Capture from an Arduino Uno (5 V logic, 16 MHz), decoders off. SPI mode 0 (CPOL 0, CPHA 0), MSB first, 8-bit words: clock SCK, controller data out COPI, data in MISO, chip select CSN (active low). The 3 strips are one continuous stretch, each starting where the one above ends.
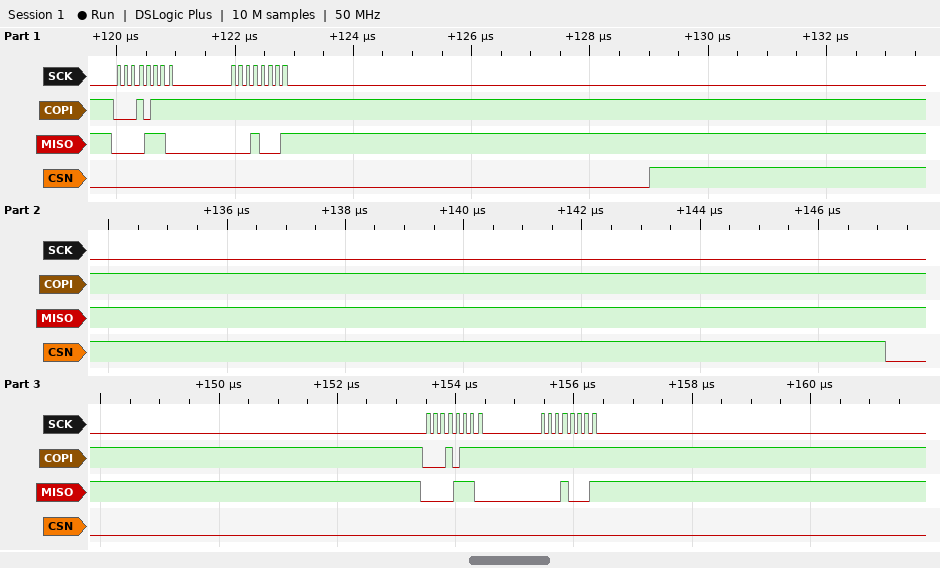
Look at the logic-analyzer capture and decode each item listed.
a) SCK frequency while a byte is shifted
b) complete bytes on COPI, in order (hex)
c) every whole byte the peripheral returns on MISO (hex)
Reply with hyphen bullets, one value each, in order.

- 8 MHz
- 17 FF 17 FF
- 0E 11 0E 11
